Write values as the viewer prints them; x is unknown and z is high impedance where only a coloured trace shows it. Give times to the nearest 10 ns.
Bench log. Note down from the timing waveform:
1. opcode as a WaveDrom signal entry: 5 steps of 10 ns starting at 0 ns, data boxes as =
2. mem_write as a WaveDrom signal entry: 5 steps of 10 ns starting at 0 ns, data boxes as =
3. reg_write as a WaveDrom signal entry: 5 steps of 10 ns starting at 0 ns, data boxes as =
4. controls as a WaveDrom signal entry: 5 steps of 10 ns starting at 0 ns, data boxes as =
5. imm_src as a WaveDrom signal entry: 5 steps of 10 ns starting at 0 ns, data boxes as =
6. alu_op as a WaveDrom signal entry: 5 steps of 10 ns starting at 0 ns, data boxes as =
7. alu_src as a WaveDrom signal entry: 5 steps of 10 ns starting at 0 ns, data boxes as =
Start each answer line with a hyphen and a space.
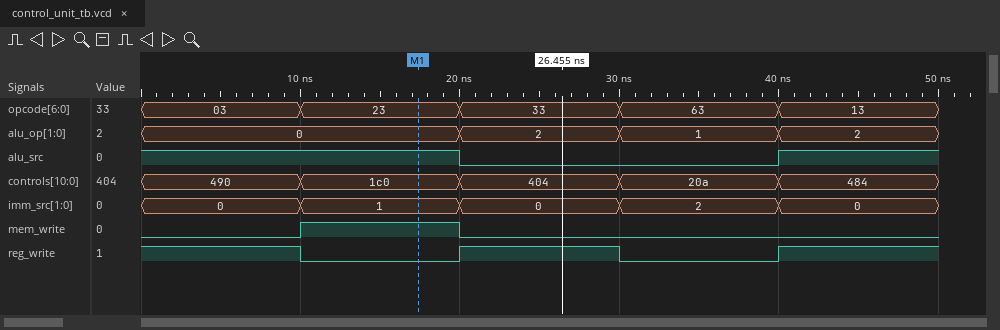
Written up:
- {name: 'opcode', wave: '=====', data: '03 23 33 63 13'}
- {name: 'mem_write', wave: '010..'}
- {name: 'reg_write', wave: '10101'}
- {name: 'controls', wave: '=====', data: '490 1c0 404 20a 484'}
- {name: 'imm_src', wave: '=====', data: '0 1 0 2 0'}
- {name: 'alu_op', wave: '=.===', data: '0 2 1 2'}
- {name: 'alu_src', wave: '1.0.1'}
